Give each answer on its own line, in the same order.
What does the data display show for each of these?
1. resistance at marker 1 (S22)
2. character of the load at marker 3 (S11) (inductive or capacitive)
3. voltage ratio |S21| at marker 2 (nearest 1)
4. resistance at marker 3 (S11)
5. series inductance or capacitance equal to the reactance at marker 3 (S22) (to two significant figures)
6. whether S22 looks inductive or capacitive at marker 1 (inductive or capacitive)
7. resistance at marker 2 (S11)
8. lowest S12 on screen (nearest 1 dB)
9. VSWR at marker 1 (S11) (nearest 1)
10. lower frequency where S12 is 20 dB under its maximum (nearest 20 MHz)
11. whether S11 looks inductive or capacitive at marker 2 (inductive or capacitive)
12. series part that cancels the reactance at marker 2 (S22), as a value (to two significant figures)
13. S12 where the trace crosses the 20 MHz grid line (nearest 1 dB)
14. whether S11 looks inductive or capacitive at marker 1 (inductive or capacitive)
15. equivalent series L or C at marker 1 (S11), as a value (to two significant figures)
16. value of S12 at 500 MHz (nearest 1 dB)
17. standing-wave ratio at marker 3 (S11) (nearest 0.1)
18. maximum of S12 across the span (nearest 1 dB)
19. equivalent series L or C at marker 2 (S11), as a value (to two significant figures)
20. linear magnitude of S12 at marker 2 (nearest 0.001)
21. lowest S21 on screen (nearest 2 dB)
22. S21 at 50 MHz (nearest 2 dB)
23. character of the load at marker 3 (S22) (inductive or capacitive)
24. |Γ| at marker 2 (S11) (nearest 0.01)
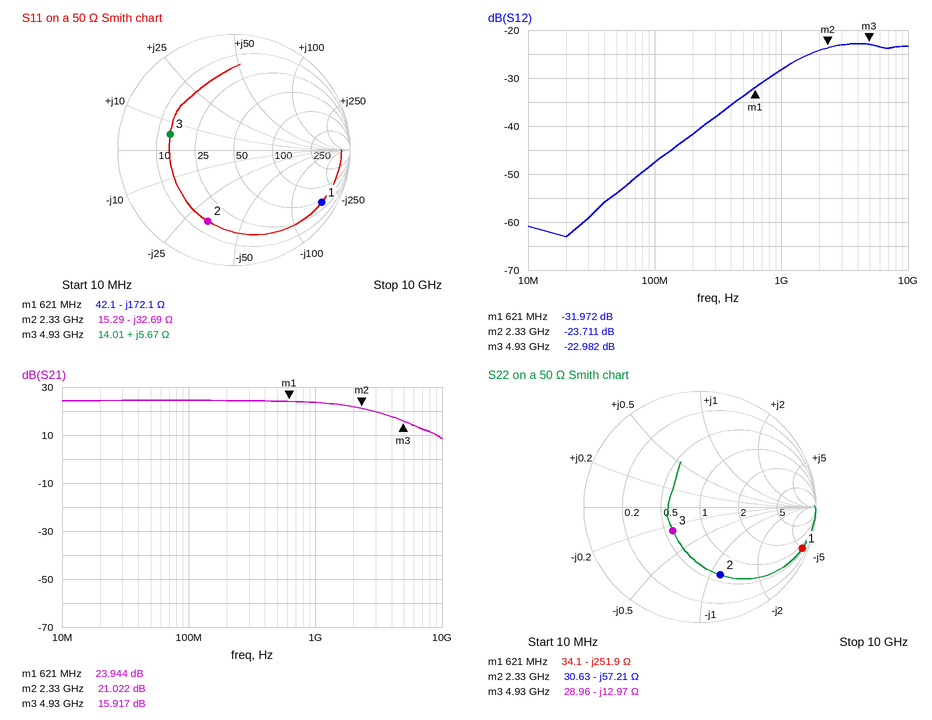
34.1 Ω
inductive
11
14.01 Ω
2.5 pF
capacitive
15.29 Ω
-63 dB
16
180 MHz
capacitive
3.9 nH
-63 dB
capacitive
1.5 pF
-34 dB
3.6
-23 dB
2.1 pF
0.065
8 dB
24 dB
capacitive
0.65
